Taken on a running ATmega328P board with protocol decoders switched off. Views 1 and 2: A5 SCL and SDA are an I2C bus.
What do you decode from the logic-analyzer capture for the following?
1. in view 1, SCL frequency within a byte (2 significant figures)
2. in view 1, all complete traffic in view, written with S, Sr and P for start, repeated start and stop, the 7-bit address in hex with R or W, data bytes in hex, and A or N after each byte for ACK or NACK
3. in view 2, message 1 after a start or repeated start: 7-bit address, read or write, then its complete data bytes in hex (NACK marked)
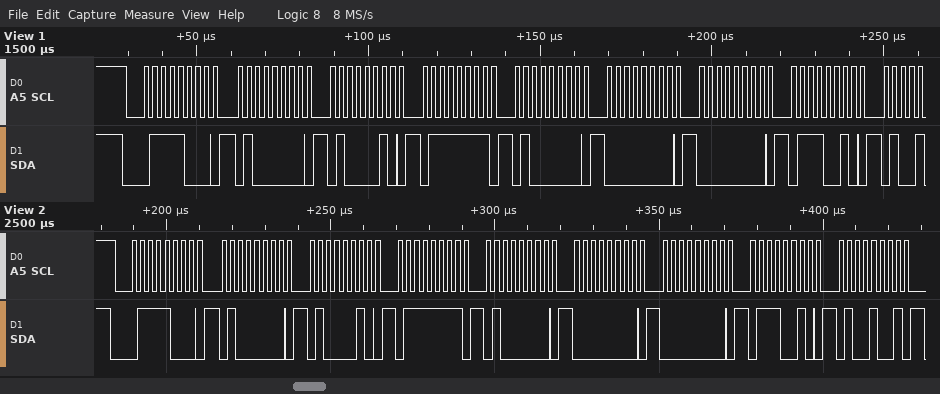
400 kHz
S 3CW A 40 A 42 A 7F A 40 A 00 A 00 A 72 A
0x3C write: 40 42 7F 40 00 00 72 49
